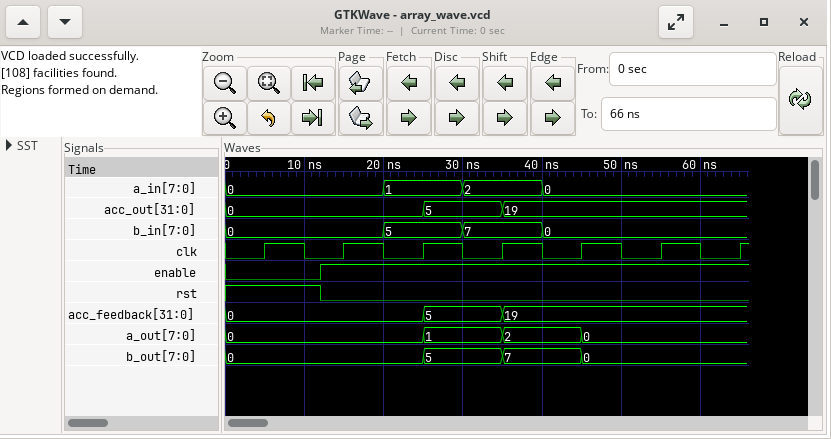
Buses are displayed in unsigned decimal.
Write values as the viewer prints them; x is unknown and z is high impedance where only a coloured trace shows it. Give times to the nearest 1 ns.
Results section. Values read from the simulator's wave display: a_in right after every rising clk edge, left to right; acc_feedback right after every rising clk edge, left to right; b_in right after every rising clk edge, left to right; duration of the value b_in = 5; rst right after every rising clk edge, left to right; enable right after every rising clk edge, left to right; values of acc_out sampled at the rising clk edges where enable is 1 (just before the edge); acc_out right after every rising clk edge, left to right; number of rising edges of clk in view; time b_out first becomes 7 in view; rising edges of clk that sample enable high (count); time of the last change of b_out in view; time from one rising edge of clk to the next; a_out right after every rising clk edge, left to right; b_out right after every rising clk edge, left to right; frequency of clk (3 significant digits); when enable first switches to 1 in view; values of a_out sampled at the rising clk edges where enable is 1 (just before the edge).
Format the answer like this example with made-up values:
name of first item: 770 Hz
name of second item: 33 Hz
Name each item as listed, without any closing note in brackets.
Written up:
a_in right after every rising clk edge, left to right: 0, 0, 1, 2, 0, 0, 0
acc_feedback right after every rising clk edge, left to right: 0, 0, 5, 19, 19, 19, 19
b_in right after every rising clk edge, left to right: 0, 0, 5, 7, 0, 0, 0
duration of the value b_in = 5: 10 ns
rst right after every rising clk edge, left to right: 1 0 0 0 0 0 0
enable right after every rising clk edge, left to right: 0 1 1 1 1 1 1
values of acc_out sampled at the rising clk edges where enable is 1: 0, 0, 5, 19, 19, 19
acc_out right after every rising clk edge, left to right: 0, 0, 5, 19, 19, 19, 19
number of rising edges of clk in view: 7
time b_out first becomes 7 in view: 35 ns
rising edges of clk that sample enable high: 6
time of the last change of b_out in view: 45 ns
time from one rising edge of clk to the next: 10 ns
a_out right after every rising clk edge, left to right: 0, 0, 1, 2, 0, 0, 0
b_out right after every rising clk edge, left to right: 0, 0, 5, 7, 0, 0, 0
frequency of clk: 100 MHz
when enable first switches to 1 in view: 12 ns
values of a_out sampled at the rising clk edges where enable is 1: 0, 0, 1, 2, 0, 0
